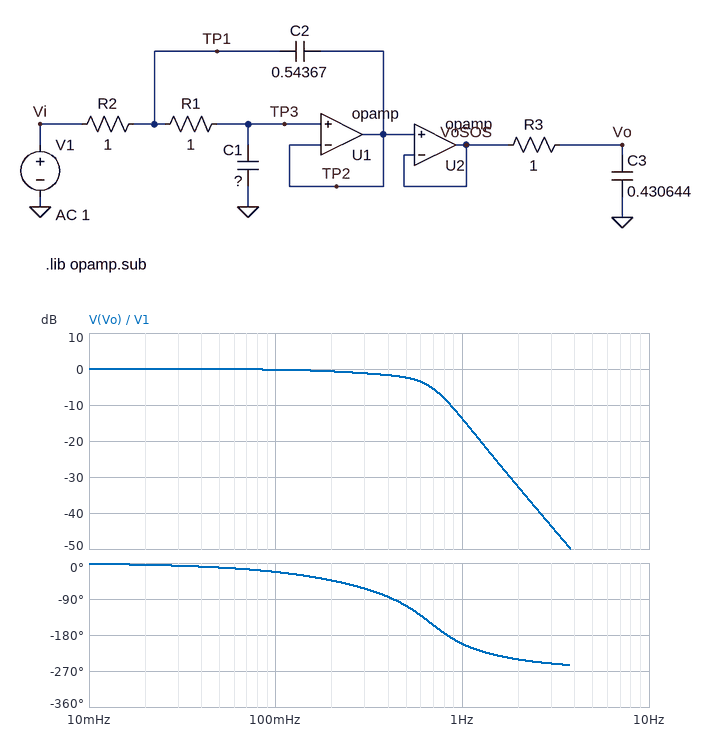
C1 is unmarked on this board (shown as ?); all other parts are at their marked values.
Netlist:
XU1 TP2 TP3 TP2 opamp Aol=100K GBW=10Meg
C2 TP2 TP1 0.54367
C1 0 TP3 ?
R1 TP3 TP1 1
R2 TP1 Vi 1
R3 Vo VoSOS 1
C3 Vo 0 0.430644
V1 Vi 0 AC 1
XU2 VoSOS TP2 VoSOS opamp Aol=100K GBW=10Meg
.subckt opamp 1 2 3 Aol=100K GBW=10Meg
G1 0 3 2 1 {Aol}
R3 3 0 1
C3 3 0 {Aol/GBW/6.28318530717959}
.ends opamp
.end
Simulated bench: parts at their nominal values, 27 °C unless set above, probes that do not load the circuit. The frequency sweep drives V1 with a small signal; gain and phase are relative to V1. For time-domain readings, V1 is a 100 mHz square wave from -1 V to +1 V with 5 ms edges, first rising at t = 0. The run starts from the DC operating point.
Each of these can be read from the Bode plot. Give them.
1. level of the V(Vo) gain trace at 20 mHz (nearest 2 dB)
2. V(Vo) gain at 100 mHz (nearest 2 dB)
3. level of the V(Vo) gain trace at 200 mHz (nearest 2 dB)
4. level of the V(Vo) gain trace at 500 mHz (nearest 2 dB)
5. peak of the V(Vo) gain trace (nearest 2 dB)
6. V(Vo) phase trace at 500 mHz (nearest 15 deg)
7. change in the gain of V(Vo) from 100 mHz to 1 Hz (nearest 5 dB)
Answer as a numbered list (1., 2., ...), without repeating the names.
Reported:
1. 0 dB
2. 0 dB
3. 0 dB
4. -2 dB
5. 0 dB
6. -105 deg
7. -15 dB
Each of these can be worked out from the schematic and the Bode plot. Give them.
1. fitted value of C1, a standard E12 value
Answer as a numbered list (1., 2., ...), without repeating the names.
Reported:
1. 100 mF
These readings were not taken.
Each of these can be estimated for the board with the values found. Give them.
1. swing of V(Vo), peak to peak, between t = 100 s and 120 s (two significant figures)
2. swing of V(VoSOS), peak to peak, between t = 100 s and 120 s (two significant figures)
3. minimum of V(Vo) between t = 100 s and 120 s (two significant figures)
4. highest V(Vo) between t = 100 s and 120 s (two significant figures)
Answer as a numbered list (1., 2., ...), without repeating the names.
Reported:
1. 2.0 V
2. 2.9 V
3. -1.0 V
4. 1.0 V
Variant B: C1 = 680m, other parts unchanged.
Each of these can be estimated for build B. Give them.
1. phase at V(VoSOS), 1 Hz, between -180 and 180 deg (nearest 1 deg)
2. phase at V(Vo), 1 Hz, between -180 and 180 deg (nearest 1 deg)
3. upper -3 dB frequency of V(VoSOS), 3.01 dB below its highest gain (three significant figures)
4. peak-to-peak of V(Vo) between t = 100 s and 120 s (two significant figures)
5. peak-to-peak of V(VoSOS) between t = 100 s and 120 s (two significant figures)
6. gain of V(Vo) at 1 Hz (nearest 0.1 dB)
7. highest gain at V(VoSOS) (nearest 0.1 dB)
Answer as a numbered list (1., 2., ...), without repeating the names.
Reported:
1. -148 deg
2. 142 deg
3. 144 mHz
4. 1.9 V
5. 2.0 V
6. -33.3 dB
7. 0 dB
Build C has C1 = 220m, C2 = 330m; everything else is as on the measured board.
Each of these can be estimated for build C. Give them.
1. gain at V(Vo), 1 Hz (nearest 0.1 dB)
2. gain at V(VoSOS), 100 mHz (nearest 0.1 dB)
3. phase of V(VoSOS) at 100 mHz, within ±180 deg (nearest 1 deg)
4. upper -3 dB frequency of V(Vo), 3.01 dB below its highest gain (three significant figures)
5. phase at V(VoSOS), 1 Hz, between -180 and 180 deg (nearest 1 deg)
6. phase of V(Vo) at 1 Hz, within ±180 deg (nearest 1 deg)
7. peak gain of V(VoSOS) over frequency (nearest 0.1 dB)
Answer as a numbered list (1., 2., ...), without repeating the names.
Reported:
1. -19.7 dB
2. -0.1 dB
3. -16 deg
4. 294 mHz
5. -124 deg
6. 166 deg
7. 0 dB
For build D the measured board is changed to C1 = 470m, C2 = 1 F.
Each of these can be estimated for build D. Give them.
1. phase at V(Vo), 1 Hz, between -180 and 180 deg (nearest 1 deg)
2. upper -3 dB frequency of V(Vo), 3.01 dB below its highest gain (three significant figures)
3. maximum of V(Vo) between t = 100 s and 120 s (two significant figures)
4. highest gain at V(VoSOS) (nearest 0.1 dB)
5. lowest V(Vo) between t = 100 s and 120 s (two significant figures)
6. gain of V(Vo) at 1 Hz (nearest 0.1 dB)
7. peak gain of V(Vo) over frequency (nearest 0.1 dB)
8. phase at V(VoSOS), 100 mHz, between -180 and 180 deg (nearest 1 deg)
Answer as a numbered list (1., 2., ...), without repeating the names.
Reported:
1. 129 deg
2. 206 mHz
3. 1.1 V
4. 0 dB
5. -1.1 V
6. -34.6 dB
7. 0 dB
8. -36 deg
